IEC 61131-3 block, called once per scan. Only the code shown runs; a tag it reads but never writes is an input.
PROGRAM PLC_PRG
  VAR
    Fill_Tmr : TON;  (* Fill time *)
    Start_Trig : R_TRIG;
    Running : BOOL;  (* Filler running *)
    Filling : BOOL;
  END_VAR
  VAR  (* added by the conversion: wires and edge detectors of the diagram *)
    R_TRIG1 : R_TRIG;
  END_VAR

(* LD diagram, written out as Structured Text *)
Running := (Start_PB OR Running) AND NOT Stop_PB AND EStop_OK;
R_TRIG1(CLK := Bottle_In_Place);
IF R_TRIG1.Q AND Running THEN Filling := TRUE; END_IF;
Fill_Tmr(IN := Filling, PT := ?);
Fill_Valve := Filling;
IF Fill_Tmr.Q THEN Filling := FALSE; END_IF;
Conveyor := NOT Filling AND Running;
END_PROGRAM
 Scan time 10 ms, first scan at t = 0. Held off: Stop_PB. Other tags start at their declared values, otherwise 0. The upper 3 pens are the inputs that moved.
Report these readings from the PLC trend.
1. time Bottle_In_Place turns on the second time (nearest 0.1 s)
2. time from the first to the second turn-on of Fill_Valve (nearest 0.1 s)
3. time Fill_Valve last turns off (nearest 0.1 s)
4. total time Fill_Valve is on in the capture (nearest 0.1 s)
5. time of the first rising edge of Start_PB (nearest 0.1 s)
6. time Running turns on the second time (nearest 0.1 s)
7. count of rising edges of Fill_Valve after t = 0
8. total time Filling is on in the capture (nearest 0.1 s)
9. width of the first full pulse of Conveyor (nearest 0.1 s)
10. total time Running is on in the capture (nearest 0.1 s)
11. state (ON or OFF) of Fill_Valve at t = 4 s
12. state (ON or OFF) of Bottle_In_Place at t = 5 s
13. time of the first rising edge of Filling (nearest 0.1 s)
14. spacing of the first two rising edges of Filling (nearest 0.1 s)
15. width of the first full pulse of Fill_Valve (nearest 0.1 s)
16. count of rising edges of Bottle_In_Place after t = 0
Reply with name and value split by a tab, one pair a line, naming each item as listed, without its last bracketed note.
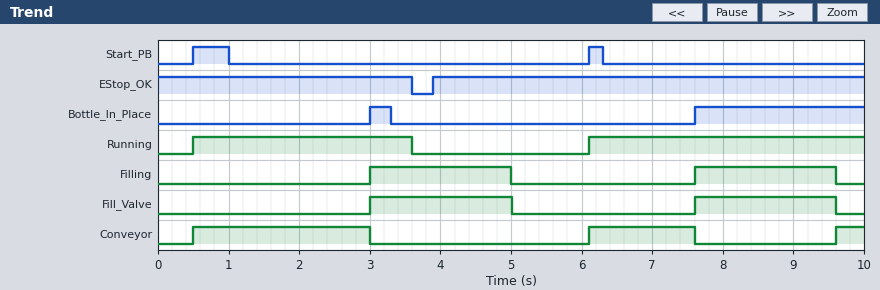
time Bottle_In_Place turns on the second time	7.6 s
time from the first to the second turn-on of Fill_Valve	4.6 s
time Fill_Valve last turns off	9.6 s
total time Fill_Valve is on in the capture	4.0 s
time of the first rising edge of Start_PB	0.5 s
time Running turns on the second time	6.1 s
count of rising edges of Fill_Valve after t = 0	2
total time Filling is on in the capture	4.0 s
width of the first full pulse of Conveyor	2.5 s
total time Running is on in the capture	7.0 s
state (ON or OFF) of Fill_Valve at t = 4 s	ON
state (ON or OFF) of Bottle_In_Place at t = 5 s	OFF
time of the first rising edge of Filling	3.0 s
spacing of the first two rising edges of Filling	4.6 s
width of the first full pulse of Fill_Valve	2.0 s
count of rising edges of Bottle_In_Place after t = 0	2
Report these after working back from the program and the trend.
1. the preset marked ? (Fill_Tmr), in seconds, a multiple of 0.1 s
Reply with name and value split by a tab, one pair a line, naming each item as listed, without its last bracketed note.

the preset marked ? (Fill_Tmr), in seconds, a multiple of 0.1 s	2.0 s
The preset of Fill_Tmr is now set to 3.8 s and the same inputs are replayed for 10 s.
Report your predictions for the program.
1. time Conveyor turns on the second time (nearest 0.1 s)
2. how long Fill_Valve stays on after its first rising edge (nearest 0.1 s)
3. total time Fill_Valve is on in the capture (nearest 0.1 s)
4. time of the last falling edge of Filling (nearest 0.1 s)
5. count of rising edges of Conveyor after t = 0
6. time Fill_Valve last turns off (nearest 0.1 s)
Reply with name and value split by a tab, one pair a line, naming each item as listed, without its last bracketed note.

time Conveyor turns on the second time	6.8 s
how long Fill_Valve stays on after its first rising edge	3.8 s
total time Fill_Valve is on in the capture	6.2 s
time of the last falling edge of Filling	6.8 s
count of rising edges of Conveyor after t = 0	2
time Fill_Valve last turns off	6.8 s
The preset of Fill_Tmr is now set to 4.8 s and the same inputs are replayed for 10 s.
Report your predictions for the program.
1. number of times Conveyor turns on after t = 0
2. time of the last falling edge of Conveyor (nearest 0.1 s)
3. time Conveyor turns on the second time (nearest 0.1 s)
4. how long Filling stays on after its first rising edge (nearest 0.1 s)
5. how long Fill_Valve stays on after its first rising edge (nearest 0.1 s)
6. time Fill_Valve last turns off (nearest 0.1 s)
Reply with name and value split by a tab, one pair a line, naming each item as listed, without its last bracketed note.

number of times Conveyor turns on after t = 0	2
time of the last falling edge of Conveyor	3.0 s
time Conveyor turns on the second time	7.8 s
how long Filling stays on after its first rising edge	4.8 s
how long Fill_Valve stays on after its first rising edge	4.8 s
time Fill_Valve last turns off	7.8 s
